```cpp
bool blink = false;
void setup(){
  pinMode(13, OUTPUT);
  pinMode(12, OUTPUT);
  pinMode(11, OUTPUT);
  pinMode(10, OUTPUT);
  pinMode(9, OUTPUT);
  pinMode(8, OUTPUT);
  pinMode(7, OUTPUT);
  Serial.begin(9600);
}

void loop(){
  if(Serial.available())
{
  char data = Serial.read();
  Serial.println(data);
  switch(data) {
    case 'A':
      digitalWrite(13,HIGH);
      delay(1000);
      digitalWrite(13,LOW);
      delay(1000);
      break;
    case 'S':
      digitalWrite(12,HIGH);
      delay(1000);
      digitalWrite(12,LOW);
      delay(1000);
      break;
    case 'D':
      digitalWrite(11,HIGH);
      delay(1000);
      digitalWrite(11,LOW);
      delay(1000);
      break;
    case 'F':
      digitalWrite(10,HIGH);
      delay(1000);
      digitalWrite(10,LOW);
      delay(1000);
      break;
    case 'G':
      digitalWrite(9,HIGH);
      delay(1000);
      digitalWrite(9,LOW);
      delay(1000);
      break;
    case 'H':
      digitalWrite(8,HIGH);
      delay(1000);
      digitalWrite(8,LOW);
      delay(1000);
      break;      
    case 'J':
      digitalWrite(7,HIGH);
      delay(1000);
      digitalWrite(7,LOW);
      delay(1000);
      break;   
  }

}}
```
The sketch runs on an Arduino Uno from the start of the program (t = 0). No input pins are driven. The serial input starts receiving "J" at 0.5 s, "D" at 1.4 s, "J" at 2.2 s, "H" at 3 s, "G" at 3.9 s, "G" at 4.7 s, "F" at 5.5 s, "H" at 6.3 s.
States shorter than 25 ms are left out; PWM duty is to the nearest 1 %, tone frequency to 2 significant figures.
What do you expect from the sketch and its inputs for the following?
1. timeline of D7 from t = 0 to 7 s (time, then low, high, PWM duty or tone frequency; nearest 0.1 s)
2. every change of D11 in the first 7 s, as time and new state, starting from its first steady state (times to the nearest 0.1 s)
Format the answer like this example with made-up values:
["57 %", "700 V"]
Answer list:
["0 s low; 0.5 s high; 1.5 s low; 4.5 s high; 5.5 s low", "0 s low; 2.5 s high; 3.5 s low"]
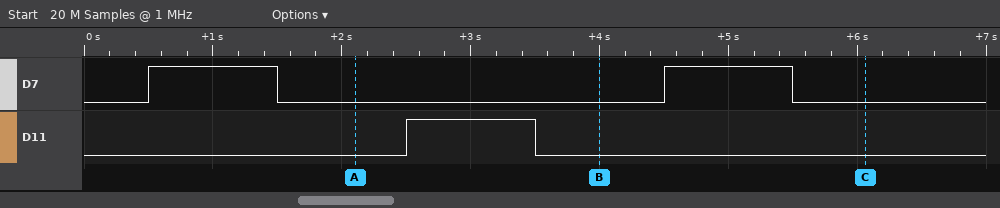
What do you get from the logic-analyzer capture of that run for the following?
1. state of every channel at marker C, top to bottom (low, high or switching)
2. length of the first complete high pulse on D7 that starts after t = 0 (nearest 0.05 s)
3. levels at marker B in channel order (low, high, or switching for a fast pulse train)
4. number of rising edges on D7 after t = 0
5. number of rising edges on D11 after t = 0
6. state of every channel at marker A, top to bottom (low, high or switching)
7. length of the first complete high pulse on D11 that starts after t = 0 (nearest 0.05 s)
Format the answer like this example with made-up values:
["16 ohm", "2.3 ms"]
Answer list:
["D7 low, D11 low", "1.00 s", "D7 low, D11 low", "2", "1", "D7 low, D11 low", "1.00 s"]
